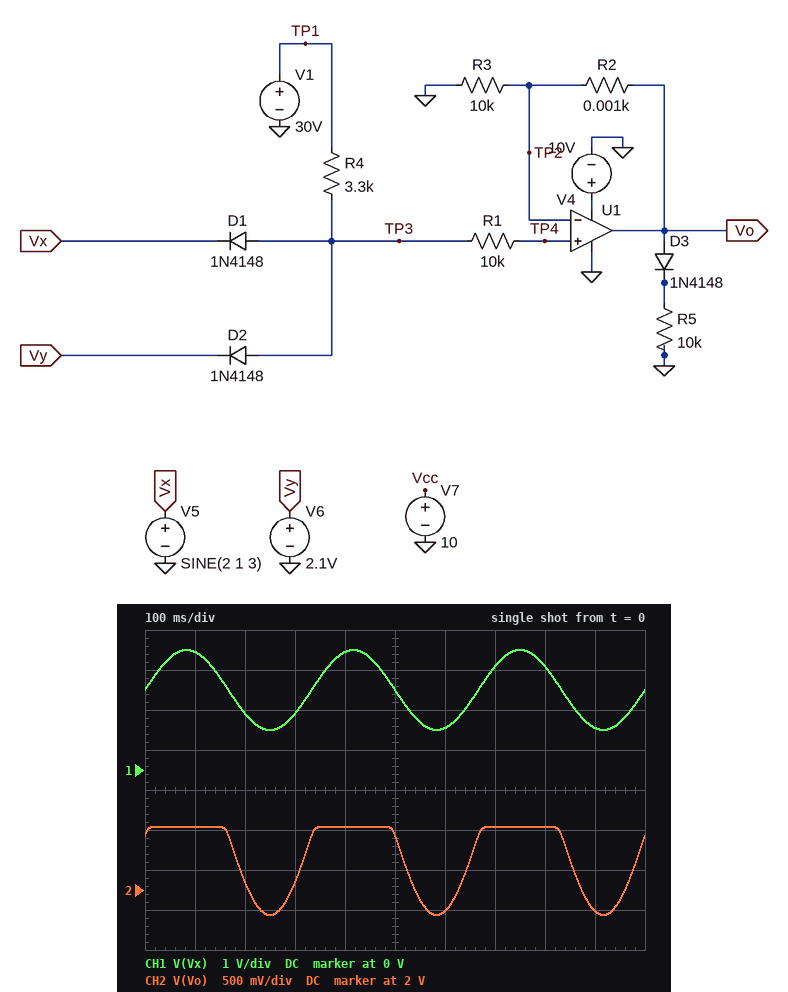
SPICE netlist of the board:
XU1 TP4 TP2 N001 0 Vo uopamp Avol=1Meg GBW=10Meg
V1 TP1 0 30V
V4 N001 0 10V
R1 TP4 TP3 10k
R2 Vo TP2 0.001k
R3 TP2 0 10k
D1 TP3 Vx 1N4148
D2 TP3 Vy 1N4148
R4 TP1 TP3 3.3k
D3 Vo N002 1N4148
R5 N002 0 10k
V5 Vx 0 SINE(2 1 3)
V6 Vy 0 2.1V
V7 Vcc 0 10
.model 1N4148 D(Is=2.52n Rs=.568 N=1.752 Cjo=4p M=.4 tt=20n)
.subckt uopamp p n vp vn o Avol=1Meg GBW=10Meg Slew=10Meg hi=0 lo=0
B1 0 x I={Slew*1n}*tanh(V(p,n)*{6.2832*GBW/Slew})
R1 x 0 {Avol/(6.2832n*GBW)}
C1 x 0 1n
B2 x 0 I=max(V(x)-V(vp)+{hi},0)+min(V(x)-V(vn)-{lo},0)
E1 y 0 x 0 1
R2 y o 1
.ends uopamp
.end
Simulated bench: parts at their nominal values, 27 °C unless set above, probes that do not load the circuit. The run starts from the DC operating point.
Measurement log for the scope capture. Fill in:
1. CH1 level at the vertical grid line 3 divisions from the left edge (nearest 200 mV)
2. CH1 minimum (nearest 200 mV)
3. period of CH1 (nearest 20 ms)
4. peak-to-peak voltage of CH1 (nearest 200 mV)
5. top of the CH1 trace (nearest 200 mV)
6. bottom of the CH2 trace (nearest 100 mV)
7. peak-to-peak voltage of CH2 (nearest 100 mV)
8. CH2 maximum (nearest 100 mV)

1.4 V
1.0 V
340 ms
2.0 V
3.0 V
1.7 V
1.1 V
2.8 V
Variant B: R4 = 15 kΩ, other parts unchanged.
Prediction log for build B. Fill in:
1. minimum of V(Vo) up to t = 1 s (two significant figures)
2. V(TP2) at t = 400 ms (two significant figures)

1.6 V
2.7 V
